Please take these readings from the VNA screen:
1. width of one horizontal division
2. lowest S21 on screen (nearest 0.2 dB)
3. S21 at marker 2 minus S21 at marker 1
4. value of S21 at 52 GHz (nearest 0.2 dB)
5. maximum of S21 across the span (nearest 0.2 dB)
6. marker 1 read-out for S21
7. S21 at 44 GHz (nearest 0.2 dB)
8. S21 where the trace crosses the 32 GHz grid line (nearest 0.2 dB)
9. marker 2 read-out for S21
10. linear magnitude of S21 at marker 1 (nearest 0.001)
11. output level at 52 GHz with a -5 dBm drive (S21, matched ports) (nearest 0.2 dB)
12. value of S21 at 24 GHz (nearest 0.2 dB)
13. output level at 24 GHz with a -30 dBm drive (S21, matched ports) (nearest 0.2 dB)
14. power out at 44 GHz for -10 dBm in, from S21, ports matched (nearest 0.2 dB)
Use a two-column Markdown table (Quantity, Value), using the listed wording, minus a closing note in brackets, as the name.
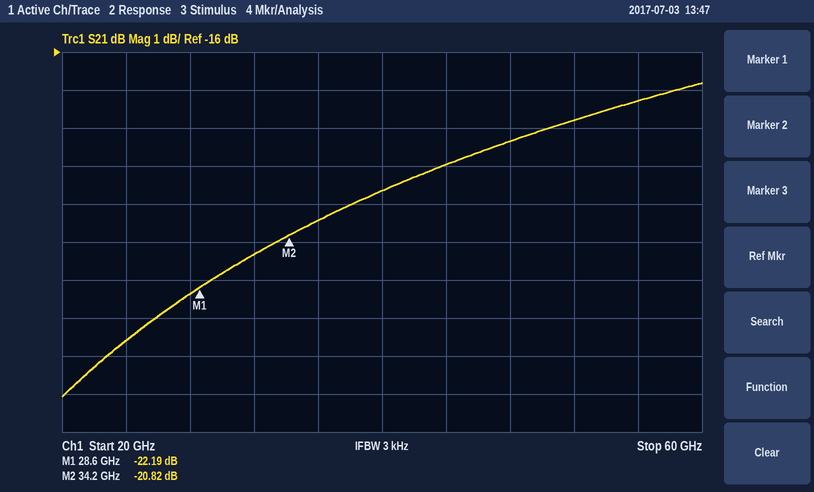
| Quantity | Value |
|---|---|
| width of one horizontal division | 4 GHz |
| lowest S21 on screen | -25.0 dB |
| S21 at marker 2 minus S21 at marker 1 | 1.37 dB |
| value of S21 at 52 GHz | -17.8 dB |
| maximum of S21 across the span | -16.8 dB |
| marker 1 read-out for S21 | -22.19 dB |
| S21 at 44 GHz | -19.0 dB |
| S21 where the trace crosses the 32 GHz grid line | -21.4 dB |
| marker 2 read-out for S21 | -20.82 dB |
| linear magnitude of S21 at marker 1 | 0.078 |
| output level at 52 GHz with a -5 dBm drive (S21, matched ports) | -22.8 dBm |
| value of S21 at 24 GHz | -23.6 dB |
| output level at 24 GHz with a -30 dBm drive (S21, matched ports) | -53.6 dBm |
| power out at 44 GHz for -10 dBm in, from S21, ports matched | -29.0 dBm |
